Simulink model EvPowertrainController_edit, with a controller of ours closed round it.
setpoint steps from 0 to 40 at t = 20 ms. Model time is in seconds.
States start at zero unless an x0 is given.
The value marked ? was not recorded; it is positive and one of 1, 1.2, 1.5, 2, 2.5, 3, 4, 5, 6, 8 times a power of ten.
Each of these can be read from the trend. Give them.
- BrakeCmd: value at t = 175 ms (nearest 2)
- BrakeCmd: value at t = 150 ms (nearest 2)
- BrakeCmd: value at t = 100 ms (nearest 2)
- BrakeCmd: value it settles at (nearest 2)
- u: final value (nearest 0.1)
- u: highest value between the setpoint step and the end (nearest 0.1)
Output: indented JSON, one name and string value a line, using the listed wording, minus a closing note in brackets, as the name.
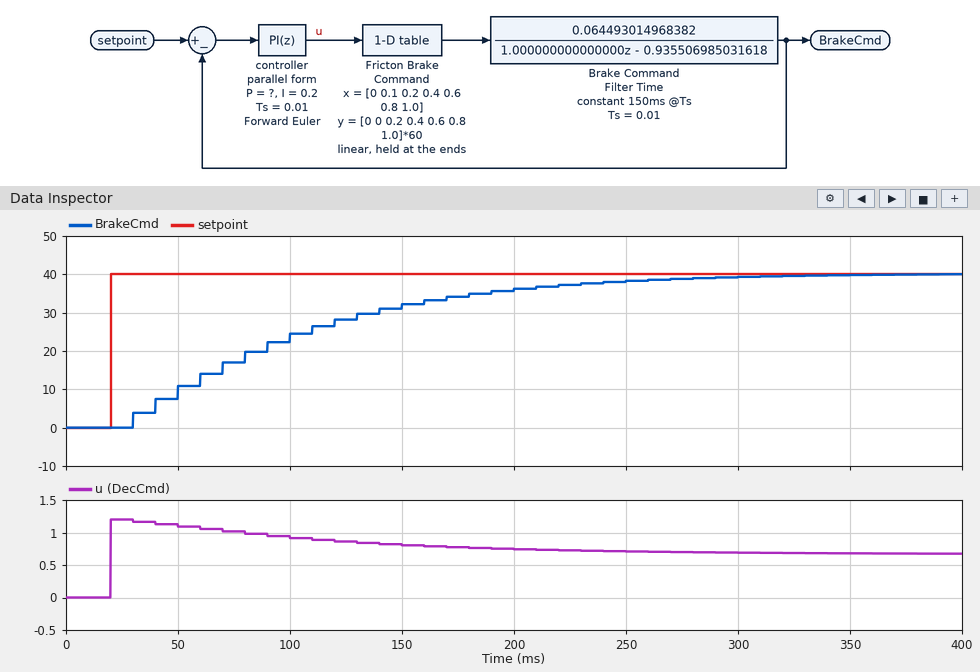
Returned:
{
  "BrakeCmd: value at t = 175 ms": "34",
  "BrakeCmd: value at t = 150 ms": "32",
  "BrakeCmd: value at t = 100 ms": "24",
  "BrakeCmd: value it settles at": "40",
  "u: final value": "0.7",
  "u: highest value between the setpoint step and the end": "1.2"
}
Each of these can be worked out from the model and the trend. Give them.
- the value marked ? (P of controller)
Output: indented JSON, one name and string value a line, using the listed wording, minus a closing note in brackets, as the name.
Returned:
{
  "the value marked ?": "0.03"
}
